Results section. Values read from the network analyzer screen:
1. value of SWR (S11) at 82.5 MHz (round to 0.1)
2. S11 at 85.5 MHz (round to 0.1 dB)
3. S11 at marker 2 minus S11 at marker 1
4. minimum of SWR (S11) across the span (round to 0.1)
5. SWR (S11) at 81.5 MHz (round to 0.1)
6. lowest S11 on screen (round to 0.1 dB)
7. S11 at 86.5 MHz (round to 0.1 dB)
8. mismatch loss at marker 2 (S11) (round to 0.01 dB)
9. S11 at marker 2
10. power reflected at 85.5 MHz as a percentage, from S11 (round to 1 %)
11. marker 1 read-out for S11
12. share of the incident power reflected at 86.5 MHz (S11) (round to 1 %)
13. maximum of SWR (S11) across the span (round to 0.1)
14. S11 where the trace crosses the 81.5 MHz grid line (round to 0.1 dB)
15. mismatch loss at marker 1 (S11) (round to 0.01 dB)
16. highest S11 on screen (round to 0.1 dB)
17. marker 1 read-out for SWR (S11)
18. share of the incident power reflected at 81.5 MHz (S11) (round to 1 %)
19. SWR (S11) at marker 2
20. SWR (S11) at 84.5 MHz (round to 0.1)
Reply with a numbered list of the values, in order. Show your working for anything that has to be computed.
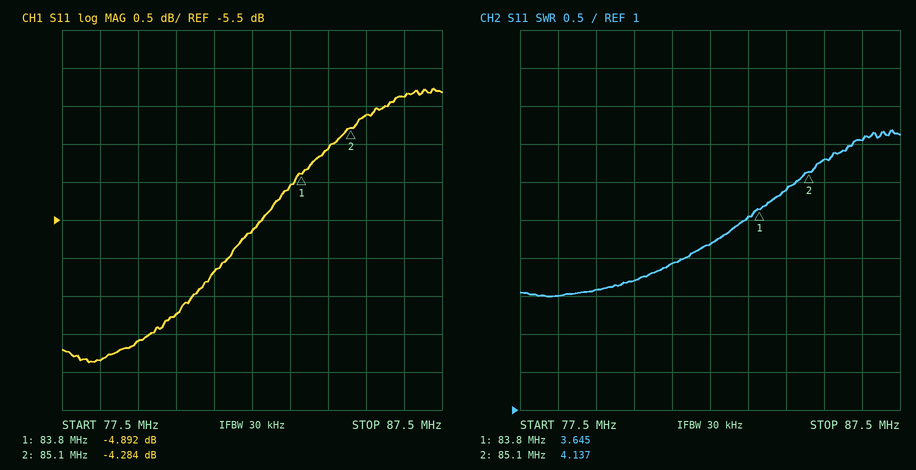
1. 3.2
2. -4.1 dB
3. -4.284 − (-4.892) = 0.608 dB
4. 2.5
5. 2.9
6. -7.4 dB
7. -3.9 dB
8. −10 log10(1 − 10^(-4.284/10)) ≈ 2.03 dB
9. -4.284 dB
10. 10^(-4.1/10) ≈ 39 %
11. -4.892 dB
12. 10^(-3.9/10) ≈ 41 %
13. 4.7
14. -6.2 dB
15. −10 log10(1 − 10^(-4.892/10)) ≈ 1.70 dB
16. -3.8 dB
17. 3.645
18. 10^(-6.2/10) ≈ 24 %
19. 4.137
20. 3.9
